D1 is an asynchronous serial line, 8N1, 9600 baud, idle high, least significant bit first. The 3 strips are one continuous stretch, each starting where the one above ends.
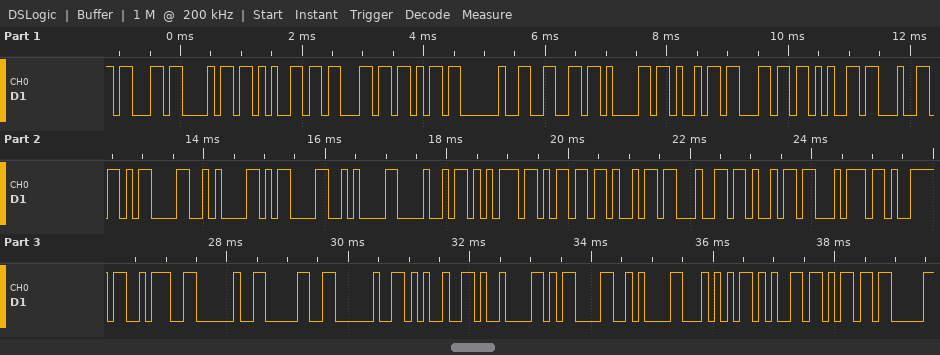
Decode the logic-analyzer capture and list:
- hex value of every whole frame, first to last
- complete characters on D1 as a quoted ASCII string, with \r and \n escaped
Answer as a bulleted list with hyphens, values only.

- 63 68 65 63 6B 20 66 61 69 6C 65 64 0D 0A 0D 0A 48 75 6D 69 64 69 74 79 3A 20 30 20 25 09 0D 0A 54 65 6D
- "check failed\r\n\r\nHumidity: 0 %\t\r\nTem"
